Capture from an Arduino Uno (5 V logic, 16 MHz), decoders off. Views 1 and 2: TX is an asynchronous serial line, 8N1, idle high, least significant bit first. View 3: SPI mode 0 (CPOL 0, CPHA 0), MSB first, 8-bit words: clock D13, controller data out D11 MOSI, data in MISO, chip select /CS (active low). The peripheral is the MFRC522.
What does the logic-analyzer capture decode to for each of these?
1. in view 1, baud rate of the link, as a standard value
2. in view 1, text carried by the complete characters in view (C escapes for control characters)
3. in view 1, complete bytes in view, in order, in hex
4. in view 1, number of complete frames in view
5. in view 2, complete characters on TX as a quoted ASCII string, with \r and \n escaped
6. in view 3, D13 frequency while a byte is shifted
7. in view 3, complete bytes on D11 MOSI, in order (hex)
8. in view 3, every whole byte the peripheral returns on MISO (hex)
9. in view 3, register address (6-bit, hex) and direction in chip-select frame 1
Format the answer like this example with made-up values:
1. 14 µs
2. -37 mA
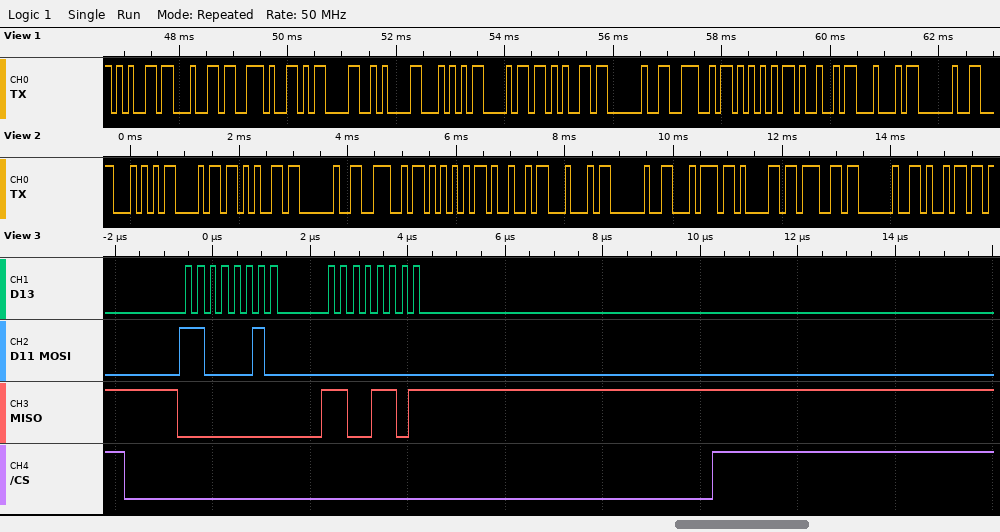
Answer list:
1. 9600 baud
2. "ed.\r\nThe NUID "
3. 65 64 2E 0D 0A 54 68 65 20 4E 55 49 44 20
4. 14
5. "The NUID tag i"
6. 4 MHz
7. C2 00
8. 00 CD
9. 0x21 read
